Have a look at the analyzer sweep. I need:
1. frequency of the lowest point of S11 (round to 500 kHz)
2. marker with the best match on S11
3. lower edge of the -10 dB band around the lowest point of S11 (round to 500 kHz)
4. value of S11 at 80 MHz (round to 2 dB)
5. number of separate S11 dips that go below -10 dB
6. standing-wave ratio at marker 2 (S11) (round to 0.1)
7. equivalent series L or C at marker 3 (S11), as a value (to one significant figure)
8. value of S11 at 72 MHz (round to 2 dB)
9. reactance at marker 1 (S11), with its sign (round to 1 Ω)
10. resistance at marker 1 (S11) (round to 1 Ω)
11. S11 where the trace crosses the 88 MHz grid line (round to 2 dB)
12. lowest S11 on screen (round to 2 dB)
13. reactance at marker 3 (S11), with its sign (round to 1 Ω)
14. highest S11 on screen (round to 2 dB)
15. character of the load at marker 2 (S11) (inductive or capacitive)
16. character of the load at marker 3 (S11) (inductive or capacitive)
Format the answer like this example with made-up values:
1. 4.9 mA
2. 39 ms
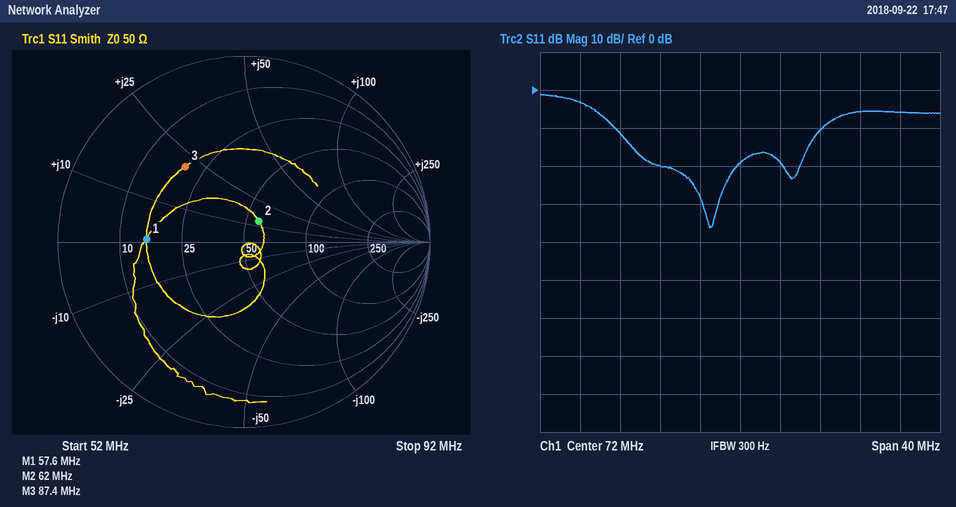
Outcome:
1. 69.0 MHz
2. marker 2
3. 59.5 MHz
4. -10 dB
5. 2
6. 1.3
7. 40 nH
8. -20 dB
9. +1 Ω
10. 16 Ω
11. -6 dB
12. -36 dB
13. +21 Ω
14. -2 dB
15. inductive
16. inductive
